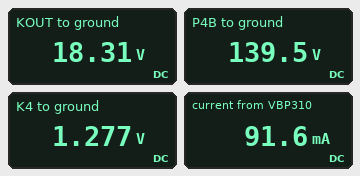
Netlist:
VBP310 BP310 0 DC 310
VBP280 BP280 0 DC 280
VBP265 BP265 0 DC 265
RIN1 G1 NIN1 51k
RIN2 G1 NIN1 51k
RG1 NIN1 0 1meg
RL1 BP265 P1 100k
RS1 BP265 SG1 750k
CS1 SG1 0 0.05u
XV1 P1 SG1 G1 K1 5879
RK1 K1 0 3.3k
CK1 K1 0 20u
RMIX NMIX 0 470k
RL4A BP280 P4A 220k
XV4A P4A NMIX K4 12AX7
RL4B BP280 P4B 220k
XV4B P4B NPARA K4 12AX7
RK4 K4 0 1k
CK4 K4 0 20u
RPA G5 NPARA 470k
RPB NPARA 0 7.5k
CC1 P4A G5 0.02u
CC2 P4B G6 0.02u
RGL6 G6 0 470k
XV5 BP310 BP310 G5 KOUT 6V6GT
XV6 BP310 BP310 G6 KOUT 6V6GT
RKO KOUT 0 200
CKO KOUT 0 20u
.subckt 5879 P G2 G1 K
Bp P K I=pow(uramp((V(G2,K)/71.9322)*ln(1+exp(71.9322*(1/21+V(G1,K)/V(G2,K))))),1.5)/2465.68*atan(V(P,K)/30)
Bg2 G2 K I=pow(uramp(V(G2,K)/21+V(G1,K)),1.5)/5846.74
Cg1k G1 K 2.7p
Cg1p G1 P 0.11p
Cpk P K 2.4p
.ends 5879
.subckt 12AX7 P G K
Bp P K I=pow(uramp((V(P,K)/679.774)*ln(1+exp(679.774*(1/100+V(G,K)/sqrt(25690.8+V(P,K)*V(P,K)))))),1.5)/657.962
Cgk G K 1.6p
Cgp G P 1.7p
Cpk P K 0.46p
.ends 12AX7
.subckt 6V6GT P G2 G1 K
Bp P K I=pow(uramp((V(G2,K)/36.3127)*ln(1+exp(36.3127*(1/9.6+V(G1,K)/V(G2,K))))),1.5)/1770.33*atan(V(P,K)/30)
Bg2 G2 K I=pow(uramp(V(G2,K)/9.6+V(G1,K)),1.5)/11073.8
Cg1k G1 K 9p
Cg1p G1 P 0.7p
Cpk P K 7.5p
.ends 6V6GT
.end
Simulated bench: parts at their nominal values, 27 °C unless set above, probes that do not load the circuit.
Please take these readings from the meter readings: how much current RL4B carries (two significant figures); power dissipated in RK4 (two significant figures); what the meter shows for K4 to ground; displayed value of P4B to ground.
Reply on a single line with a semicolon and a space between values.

640 µA; 1.6 mW; 1.277 V; 139.5 V
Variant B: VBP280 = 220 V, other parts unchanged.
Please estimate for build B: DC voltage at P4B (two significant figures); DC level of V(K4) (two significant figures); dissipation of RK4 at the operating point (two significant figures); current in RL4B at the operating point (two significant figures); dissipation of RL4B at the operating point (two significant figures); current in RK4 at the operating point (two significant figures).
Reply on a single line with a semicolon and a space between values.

110 V; 1.0 V; 1.1 mW; 520 µA; 59 mW; 1.0 mA
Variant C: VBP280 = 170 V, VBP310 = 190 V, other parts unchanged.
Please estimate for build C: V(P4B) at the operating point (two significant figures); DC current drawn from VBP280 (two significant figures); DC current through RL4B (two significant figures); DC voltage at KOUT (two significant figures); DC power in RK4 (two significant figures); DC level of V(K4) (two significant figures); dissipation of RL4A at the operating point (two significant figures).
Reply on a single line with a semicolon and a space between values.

79 V; 830 µA; 410 µA; 10 V; 690 µW; 830 mV; 38 mW
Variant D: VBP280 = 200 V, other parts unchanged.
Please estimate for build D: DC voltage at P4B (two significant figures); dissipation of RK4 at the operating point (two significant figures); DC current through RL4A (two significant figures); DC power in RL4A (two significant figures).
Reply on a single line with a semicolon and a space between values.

95 V; 910 µW; 480 µA; 50 mW
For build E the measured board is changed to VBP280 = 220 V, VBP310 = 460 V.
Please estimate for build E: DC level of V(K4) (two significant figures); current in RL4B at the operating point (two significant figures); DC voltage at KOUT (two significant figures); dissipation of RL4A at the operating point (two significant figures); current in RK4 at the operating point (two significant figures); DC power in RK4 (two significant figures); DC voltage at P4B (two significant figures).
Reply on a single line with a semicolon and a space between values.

1.0 V; 520 µA; 29 V; 59 mW; 1.0 mA; 1.1 mW; 110 V
